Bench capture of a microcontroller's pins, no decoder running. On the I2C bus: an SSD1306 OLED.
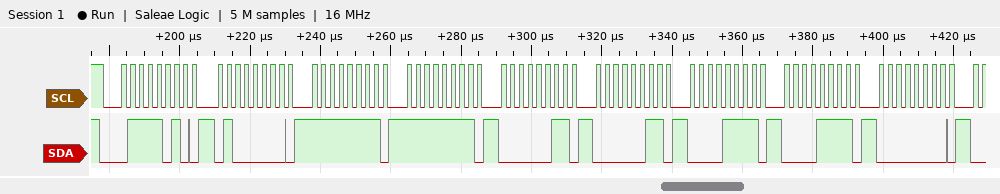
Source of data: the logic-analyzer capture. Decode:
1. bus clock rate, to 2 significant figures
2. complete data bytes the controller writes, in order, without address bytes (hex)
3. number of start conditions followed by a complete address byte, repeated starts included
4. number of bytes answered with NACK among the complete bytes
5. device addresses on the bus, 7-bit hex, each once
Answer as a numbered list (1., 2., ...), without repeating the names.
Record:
1. 400 kHz
2. 40 FF FF 03 03 0F 0F 00
3. 1
4. 0
5. 0x3D
